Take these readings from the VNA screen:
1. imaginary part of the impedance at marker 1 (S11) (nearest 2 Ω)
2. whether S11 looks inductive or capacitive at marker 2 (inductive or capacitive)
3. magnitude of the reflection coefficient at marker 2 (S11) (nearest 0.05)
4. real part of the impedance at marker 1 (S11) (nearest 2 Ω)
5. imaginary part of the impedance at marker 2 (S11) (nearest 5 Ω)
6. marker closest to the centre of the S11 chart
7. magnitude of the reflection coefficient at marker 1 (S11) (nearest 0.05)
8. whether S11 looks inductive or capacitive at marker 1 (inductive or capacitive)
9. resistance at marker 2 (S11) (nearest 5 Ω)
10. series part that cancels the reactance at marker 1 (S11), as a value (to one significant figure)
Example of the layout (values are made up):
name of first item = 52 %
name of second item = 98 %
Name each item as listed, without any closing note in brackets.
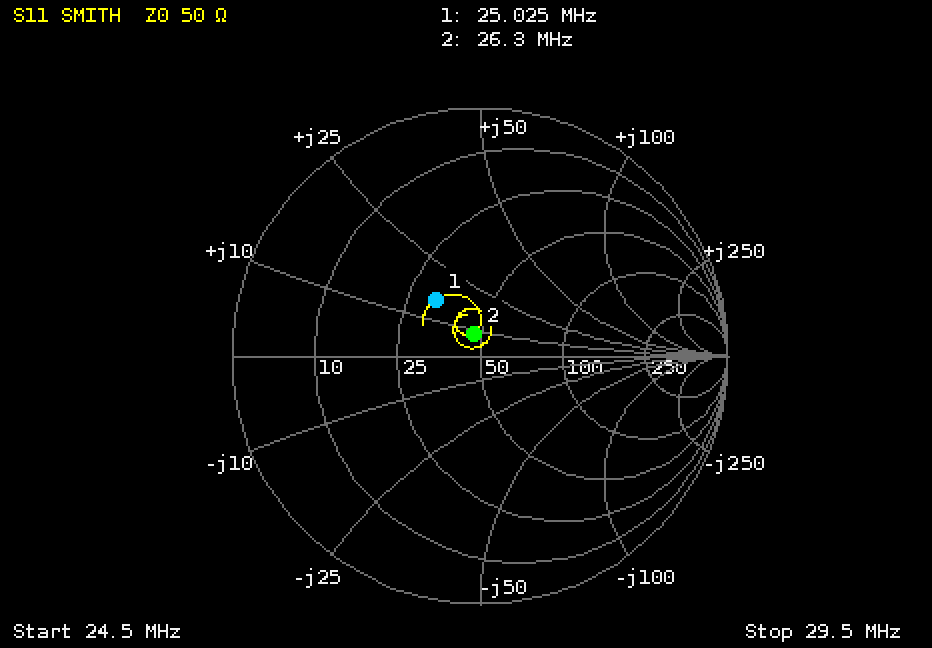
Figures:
imaginary part of the impedance at marker 1 (S11) = +16 Ω
whether S11 looks inductive or capacitive at marker 2 = inductive
magnitude of the reflection coefficient at marker 2 (S11) = 0.10
real part of the impedance at marker 1 (S11) = 32 Ω
imaginary part of the impedance at marker 2 (S11) = +10 Ω
marker closest to the centre of the S11 chart = marker 2
magnitude of the reflection coefficient at marker 1 (S11) = 0.30
whether S11 looks inductive or capacitive at marker 1 = inductive
resistance at marker 2 (S11) = 45 Ω
series part that cancels the reactance at marker 1 (S11), as a value = 400 pF
